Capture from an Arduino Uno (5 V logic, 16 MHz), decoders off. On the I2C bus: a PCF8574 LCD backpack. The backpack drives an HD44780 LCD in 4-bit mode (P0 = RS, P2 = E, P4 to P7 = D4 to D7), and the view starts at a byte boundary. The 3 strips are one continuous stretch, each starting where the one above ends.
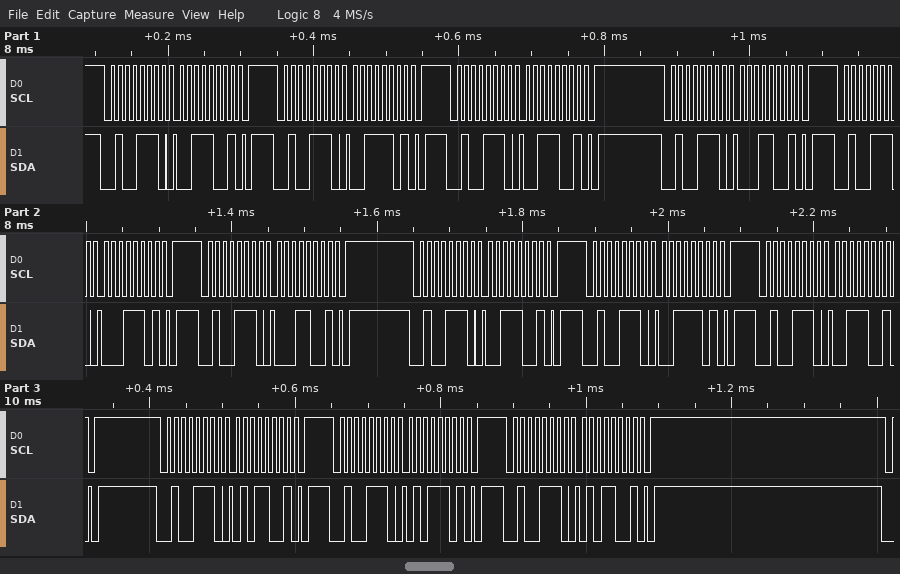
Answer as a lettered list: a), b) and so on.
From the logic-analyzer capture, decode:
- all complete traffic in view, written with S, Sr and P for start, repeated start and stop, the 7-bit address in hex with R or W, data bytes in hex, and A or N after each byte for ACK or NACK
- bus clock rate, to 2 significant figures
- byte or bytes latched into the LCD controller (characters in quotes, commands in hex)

a) S 27W A 39 A P S 27W A 3D A P S 27W A 39 A P S 27W A 19 A P S 27W A 1D A P S 27W A 19 A P S 27W A 39 A P S 27W A 3D A P S 27W A 39 A P S 27W A 59 A P S 27W A 5D A P S 27W A 59 A P
b) 100 kHz
c) '1' '5'
